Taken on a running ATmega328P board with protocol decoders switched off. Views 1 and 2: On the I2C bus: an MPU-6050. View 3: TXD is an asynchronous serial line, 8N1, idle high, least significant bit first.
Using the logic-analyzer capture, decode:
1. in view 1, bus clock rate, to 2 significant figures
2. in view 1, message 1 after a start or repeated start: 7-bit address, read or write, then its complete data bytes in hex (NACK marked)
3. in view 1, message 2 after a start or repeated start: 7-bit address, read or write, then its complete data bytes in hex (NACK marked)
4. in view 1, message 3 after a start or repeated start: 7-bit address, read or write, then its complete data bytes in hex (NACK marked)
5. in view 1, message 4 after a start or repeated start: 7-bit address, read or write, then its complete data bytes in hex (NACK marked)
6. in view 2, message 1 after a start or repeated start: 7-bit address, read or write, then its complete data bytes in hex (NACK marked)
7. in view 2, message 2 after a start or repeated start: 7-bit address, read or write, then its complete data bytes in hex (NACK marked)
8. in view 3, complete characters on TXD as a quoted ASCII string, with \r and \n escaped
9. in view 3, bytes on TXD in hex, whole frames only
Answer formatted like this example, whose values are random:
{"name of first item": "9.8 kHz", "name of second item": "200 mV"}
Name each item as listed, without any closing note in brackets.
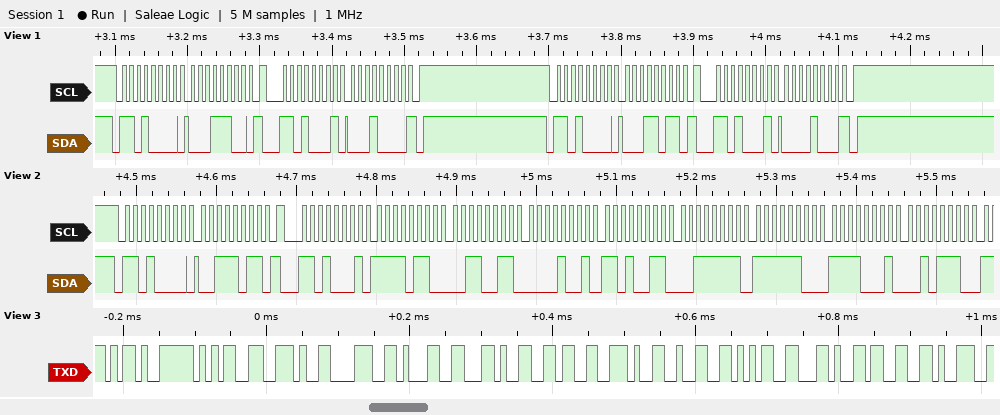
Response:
{"in view 1, bus clock rate, to 2 significant figures": "100 kHz", "in view 1, message 1 after a start or repeated start: 7-bit address, read or write, then its complete data bytes in hex": "0x68 write: 1C", "in view 1, message 2 after a start or repeated start: 7-bit address, read or write, then its complete data bytes in hex": "0x68 read: 10 NACK", "in view 1, message 3 after a start or repeated start: 7-bit address, read or write, then its complete data bytes in hex": "0x68 write: 1B", "in view 1, message 4 after a start or repeated start: 7-bit address, read or write, then its complete data bytes in hex": "0x68 read: 08 NACK", "in view 2, message 1 after a start or repeated start: 7-bit address, read or write, then its complete data bytes in hex": "0x68 write: 3B", "in view 2, message 2 after a start or repeated start: 7-bit address, read or write, then its complete data bytes in hex": "0x68 read: F6 33 09 D3 3F FC F1 2E", "in view 3, complete characters on TXD as a quoted ASCII string, with \\r and \\n escaped": "\"-5.81,6.25,39\"", "in view 3, bytes on TXD in hex, whole frames only": "2D 35 2E 38 31 2C 36 2E 32 35 2C 33 39"}
